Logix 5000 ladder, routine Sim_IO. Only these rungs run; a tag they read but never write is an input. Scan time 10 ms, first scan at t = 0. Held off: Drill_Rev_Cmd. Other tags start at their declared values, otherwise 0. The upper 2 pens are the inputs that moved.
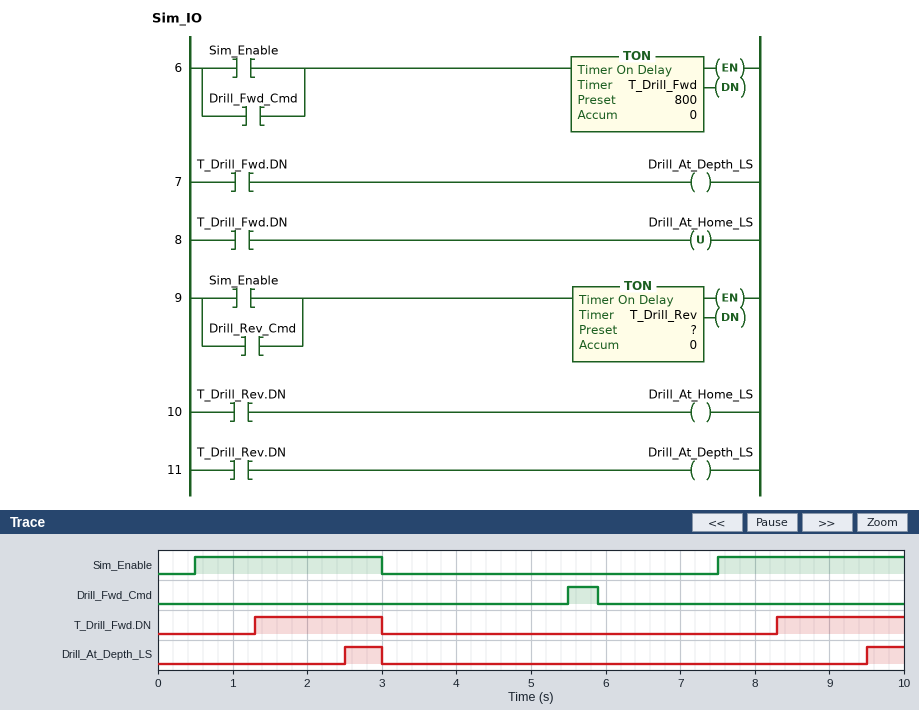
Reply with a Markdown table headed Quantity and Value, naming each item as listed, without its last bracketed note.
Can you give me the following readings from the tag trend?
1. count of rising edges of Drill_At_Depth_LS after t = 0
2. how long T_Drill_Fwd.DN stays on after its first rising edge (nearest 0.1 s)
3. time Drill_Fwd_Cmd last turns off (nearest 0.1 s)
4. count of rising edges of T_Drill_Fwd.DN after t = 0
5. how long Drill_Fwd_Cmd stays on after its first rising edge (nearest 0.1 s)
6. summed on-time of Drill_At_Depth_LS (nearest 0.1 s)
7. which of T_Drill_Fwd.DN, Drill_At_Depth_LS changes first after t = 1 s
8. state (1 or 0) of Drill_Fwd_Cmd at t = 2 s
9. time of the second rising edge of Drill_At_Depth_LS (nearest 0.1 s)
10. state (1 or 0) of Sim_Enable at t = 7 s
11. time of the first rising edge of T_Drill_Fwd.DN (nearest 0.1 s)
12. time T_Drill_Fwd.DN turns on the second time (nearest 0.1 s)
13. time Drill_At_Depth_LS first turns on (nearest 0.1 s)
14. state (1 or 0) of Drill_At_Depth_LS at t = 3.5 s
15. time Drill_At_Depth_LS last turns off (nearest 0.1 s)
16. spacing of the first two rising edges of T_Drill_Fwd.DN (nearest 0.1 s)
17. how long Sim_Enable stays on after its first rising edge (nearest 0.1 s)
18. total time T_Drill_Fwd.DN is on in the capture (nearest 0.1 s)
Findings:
| Quantity | Value |
|---|---|
| count of rising edges of Drill_At_Depth_LS after t = 0 | 2 |
| how long T_Drill_Fwd.DN stays on after its first rising edge | 1.7 s |
| time Drill_Fwd_Cmd last turns off | 5.9 s |
| count of rising edges of T_Drill_Fwd.DN after t = 0 | 2 |
| how long Drill_Fwd_Cmd stays on after its first rising edge | 0.4 s |
| summed on-time of Drill_At_Depth_LS | 1.0 s |
| which of T_Drill_Fwd.DN, Drill_At_Depth_LS changes first after t = 1 s | T_Drill_Fwd.DN |
| state (1 or 0) of Drill_Fwd_Cmd at t = 2 s | 0 |
| time of the second rising edge of Drill_At_Depth_LS | 9.5 s |
| state (1 or 0) of Sim_Enable at t = 7 s | 0 |
| time of the first rising edge of T_Drill_Fwd.DN | 1.3 s |
| time T_Drill_Fwd.DN turns on the second time | 8.3 s |
| time Drill_At_Depth_LS first turns on | 2.5 s |
| state (1 or 0) of Drill_At_Depth_LS at t = 3.5 s | 0 |
| time Drill_At_Depth_LS last turns off | 3.0 s |
| spacing of the first two rising edges of T_Drill_Fwd.DN | 7.0 s |
| how long Sim_Enable stays on after its first rising edge | 2.5 s |
| total time T_Drill_Fwd.DN is on in the capture | 3.4 s |
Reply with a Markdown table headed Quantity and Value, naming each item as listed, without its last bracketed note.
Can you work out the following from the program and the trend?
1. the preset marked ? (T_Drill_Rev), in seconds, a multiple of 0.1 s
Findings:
| Quantity | Value |
|---|---|
| the preset marked ? (T_Drill_Rev), in seconds, a multiple of 0.1 s | 2.0 s |
